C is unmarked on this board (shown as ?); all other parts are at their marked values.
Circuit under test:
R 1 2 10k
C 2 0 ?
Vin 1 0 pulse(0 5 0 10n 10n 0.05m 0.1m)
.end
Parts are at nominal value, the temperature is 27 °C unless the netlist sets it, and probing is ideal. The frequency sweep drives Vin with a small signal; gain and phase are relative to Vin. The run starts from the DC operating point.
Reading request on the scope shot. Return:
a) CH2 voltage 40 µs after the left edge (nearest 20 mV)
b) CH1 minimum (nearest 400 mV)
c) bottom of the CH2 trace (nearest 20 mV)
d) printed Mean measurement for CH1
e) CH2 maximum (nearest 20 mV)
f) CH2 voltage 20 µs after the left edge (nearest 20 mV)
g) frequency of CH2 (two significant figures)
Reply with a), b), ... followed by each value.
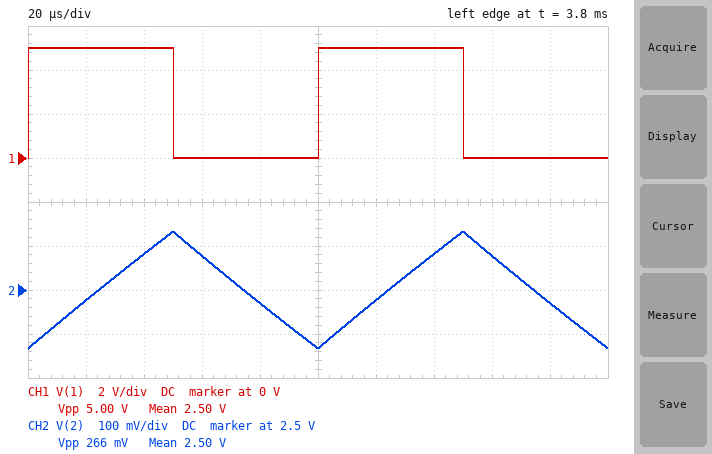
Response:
a) 2.58 V
b) 0 V
c) 2.36 V
d) 2.50 V
e) 2.64 V
f) 2.48 V
g) 10 kHz
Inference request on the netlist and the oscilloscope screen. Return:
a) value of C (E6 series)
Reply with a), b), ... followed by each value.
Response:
a) 47 nF
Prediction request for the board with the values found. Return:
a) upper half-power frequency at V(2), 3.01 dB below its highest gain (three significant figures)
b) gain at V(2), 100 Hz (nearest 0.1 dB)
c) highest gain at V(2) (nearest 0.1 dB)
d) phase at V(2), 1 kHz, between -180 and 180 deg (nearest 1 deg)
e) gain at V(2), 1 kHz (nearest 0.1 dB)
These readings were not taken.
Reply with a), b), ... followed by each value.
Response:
a) 339 Hz
b) -0.4 dB
c) 0 dB
d) -71 deg
e) -9.9 dB
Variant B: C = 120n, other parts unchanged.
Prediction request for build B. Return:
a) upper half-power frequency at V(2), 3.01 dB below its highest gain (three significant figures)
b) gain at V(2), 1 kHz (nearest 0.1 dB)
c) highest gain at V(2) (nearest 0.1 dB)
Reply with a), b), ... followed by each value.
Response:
a) 133 Hz
b) -17.6 dB
c) 0 dB
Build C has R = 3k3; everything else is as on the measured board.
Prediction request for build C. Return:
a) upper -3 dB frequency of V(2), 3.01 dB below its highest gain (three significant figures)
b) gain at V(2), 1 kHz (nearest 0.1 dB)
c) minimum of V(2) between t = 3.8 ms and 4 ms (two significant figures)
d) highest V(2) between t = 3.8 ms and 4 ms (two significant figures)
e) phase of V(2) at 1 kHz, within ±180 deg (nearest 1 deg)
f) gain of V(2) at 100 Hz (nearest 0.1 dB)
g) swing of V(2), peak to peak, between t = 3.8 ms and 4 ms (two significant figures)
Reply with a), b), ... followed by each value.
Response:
a) 1.03 kHz
b) -2.9 dB
c) 2.1 V
d) 2.9 V
e) -44 deg
f) 0 dB
g) 800 mV
